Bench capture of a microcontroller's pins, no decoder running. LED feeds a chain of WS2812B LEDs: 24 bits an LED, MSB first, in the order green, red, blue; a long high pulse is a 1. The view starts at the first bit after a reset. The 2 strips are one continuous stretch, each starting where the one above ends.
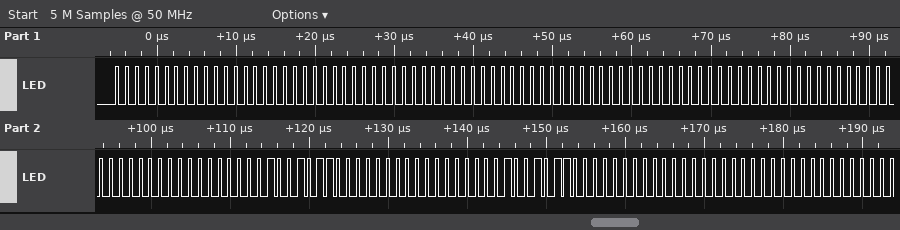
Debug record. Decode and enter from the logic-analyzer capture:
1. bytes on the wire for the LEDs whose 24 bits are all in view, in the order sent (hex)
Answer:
00 00 00 00 00 00 00 00 00 00 00 00 96 00 00 96 00 00
